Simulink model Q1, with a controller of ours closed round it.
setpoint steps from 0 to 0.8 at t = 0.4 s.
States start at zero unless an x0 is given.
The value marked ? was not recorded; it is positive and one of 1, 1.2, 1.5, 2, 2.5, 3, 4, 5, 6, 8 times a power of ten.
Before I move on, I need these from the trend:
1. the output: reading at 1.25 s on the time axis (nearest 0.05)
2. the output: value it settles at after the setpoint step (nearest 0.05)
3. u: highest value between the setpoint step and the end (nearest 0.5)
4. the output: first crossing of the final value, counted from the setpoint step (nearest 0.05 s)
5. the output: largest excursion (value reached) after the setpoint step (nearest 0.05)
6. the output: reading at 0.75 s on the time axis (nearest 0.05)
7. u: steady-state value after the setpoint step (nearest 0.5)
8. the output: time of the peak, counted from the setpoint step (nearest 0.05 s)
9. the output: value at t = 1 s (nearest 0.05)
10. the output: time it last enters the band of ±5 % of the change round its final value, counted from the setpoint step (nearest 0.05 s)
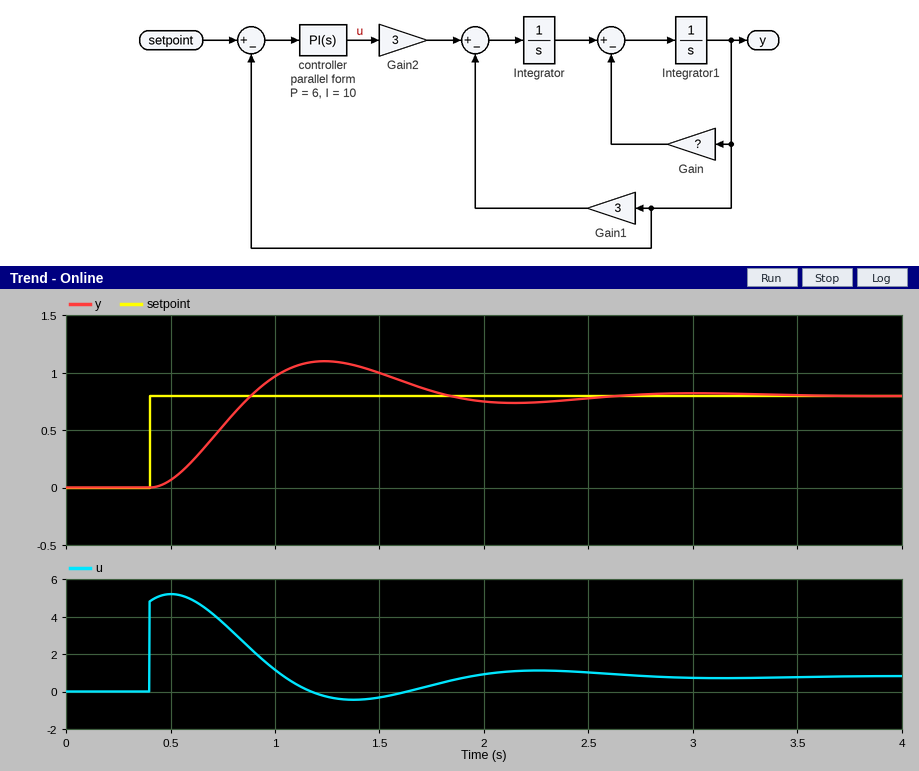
1.10
0.80
5.0
0.50 s
1.10
0.55
1.0
0.85 s
0.95
2.00 s
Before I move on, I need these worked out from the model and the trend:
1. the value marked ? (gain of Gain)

5
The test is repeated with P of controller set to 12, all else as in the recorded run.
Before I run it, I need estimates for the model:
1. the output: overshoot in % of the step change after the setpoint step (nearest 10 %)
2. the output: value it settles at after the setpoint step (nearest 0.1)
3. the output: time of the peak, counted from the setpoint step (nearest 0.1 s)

30 %
0.8
0.6 s
